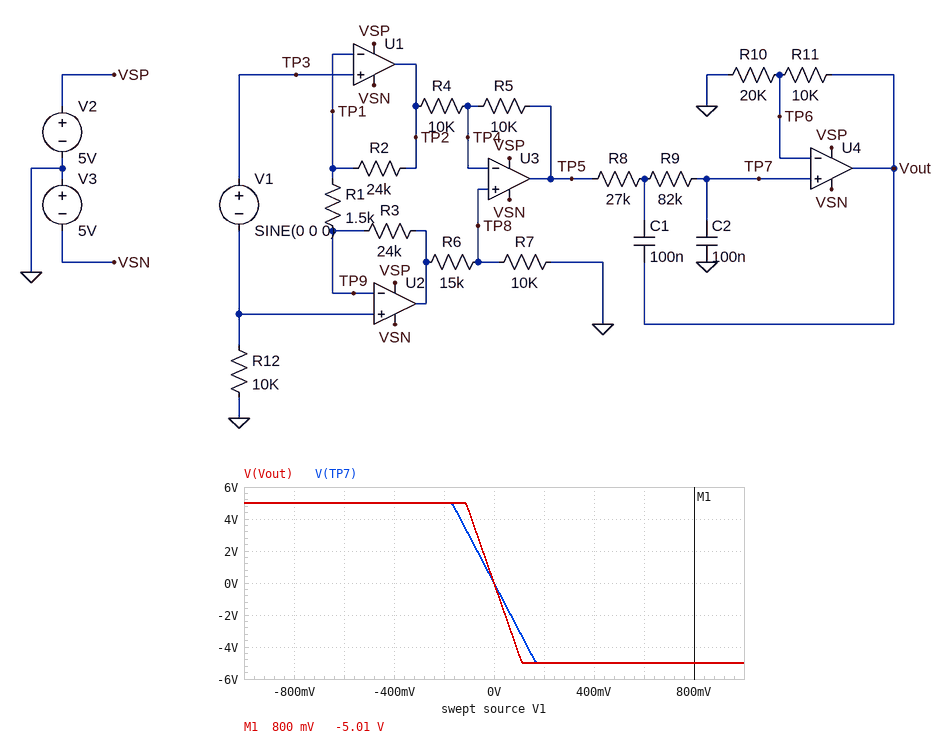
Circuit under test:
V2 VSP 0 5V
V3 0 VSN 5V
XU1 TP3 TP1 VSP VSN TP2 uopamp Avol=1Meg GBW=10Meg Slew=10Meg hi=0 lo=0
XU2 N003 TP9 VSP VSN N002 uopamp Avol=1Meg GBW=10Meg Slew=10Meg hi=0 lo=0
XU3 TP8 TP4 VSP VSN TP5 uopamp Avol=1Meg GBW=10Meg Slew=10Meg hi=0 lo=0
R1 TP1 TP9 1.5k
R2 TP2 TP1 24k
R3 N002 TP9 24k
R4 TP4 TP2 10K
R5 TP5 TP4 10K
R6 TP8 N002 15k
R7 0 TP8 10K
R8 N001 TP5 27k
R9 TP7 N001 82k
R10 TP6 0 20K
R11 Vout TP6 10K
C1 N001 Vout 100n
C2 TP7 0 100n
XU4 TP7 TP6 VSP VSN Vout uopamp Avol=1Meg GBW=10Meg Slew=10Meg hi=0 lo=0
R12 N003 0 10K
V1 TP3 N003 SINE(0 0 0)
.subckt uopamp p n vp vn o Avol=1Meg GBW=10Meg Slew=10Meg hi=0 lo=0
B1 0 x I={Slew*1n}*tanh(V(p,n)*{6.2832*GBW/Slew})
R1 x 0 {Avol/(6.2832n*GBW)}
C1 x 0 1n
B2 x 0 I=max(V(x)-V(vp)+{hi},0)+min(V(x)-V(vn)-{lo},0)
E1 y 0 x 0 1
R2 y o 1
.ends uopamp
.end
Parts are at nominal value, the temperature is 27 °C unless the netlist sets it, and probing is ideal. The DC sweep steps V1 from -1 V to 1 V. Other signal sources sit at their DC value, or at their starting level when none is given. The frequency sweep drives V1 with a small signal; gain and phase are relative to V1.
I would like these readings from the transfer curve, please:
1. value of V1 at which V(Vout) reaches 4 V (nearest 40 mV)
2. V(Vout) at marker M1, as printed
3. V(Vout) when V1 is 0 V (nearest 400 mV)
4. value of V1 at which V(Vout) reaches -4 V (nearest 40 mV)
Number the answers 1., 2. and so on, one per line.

1. -80 mV
2. -5.01 V
3. 0 V
4. 80 mV
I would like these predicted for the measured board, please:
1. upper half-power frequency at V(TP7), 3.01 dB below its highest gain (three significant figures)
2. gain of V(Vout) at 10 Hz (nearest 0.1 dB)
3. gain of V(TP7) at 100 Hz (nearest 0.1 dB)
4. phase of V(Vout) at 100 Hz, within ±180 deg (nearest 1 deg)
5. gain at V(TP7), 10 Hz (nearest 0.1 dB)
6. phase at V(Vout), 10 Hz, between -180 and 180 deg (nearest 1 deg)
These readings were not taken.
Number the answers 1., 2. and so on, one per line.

1. 21.3 Hz
2. 32.2 dB
3. 9.7 dB
4. 38 deg
5. 28.7 dB
6. 147 deg
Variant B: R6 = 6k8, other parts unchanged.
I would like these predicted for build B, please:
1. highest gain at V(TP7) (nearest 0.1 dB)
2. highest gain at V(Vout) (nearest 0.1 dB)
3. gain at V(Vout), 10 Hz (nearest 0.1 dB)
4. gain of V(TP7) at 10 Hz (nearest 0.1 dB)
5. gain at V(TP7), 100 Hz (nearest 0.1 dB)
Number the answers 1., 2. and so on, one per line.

1. 31.1 dB
2. 34.7 dB
3. 33.9 dB
4. 30.4 dB
5. 11.3 dB
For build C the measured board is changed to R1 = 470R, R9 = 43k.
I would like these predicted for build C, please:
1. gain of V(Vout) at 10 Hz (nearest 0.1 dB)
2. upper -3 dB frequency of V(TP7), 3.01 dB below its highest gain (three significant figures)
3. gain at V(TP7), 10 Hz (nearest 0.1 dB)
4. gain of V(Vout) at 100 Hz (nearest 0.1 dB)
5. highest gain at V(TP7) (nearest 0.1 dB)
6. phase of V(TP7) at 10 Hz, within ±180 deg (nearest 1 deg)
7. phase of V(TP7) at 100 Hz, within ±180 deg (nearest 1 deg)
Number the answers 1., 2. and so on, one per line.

1. 42.7 dB
2. 38.9 Hz
3. 39.2 dB
4. 28.8 dB
5. 39.4 dB
6. 160 deg
7. 45 deg
